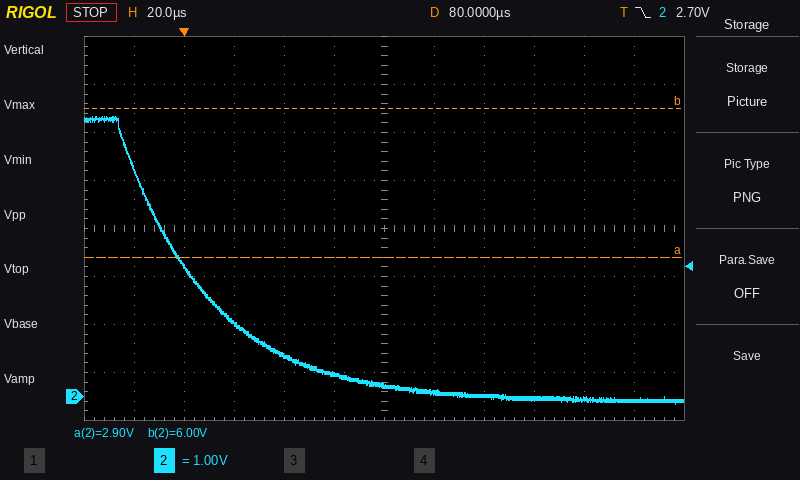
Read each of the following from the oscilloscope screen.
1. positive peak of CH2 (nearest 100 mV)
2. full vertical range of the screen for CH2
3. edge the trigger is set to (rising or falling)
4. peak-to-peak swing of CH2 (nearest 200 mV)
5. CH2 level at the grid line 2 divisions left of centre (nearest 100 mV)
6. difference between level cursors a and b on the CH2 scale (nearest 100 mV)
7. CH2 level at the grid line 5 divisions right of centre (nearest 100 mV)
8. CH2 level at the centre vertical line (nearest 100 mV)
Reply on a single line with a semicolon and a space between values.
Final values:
5.8 V; 8 V; falling; 6.0 V; 900 mV; 3.1 V; -100 mV; 200 mV
